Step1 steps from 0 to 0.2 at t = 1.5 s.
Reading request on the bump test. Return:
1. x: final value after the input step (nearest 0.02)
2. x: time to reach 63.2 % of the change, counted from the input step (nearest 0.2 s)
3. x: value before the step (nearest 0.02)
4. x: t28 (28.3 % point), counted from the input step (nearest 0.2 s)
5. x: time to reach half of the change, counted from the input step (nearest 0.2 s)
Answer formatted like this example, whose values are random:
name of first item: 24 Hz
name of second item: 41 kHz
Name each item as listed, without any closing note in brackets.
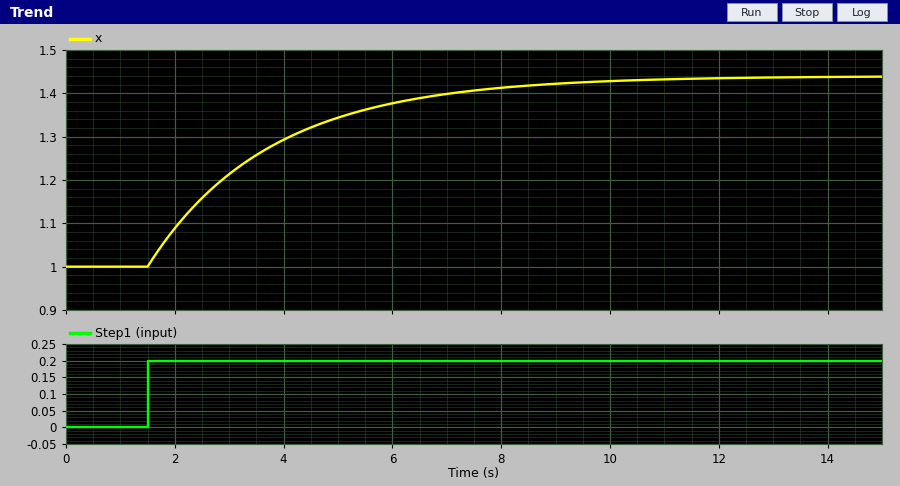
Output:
x: final value after the input step: 1.44
x: time to reach 63.2 % of the change, counted from the input step: 2.2 s
x: value before the step: 1.00
x: t28 (28.3 % point), counted from the input step: 0.8 s
x: time to reach half of the change, counted from the input step: 1.6 s
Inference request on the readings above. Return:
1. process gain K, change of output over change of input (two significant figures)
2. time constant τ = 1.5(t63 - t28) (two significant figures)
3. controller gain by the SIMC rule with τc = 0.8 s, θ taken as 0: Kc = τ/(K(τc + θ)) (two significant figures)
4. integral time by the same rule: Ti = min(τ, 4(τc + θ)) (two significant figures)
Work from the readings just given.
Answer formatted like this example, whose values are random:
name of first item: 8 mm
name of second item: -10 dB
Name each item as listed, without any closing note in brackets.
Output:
process gain K, change of output over change of input: 2.2
time constant τ = 1.5(t63 - t28): 2.1 s
controller gain by the SIMC rule with τc = 0.8 s, θ taken as 0: Kc = τ/(K(τc + θ)): 1.2
integral time by the same rule: Ti = min(τ, 4(τc + θ)): 2.1 s
